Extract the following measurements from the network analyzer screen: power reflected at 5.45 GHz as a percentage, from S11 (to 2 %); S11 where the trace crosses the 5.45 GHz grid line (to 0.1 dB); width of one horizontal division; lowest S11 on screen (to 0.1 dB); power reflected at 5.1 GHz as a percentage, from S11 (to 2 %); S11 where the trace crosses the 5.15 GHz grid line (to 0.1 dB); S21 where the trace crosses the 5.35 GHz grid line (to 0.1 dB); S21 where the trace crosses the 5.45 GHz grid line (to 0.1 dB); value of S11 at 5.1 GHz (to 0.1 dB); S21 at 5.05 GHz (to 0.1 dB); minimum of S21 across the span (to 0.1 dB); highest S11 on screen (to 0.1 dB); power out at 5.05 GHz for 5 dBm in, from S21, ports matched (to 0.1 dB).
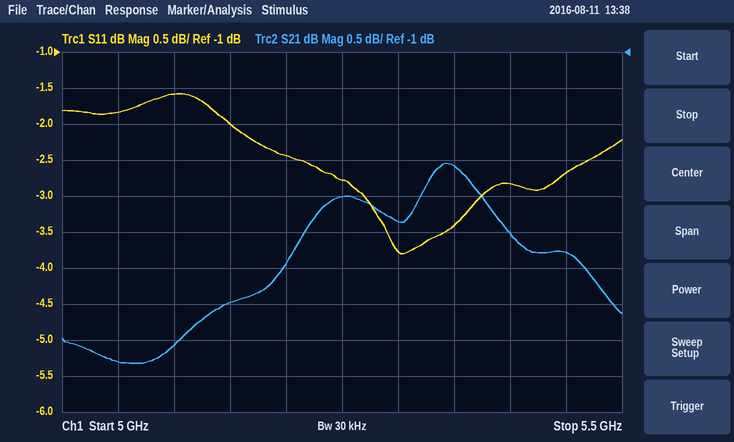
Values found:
54 %
-2.7 dB
50 MHz
-3.8 dB
70 %
-2.0 dB
-2.6 dB
-3.8 dB
-1.6 dB
-5.3 dB
-5.3 dB
-1.6 dB
-0.3 dBm
